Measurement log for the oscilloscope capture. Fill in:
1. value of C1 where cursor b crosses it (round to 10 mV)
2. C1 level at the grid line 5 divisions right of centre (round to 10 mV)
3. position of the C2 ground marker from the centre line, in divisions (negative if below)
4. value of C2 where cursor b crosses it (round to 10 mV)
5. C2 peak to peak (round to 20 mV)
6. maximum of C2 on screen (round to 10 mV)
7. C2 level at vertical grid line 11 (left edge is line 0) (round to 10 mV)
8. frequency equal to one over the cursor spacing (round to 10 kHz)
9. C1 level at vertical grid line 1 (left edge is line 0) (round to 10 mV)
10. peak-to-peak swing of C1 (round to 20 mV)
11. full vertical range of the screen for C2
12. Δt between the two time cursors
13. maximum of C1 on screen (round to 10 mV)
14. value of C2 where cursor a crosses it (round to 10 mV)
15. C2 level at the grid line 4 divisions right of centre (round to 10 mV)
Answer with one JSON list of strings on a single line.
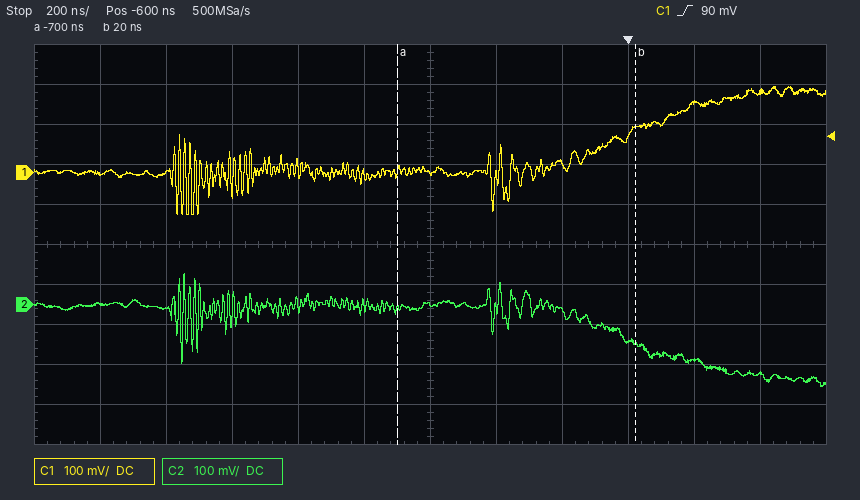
["110 mV", "200 mV", "-1.5 div", "-100 mV", "280 mV", "80 mV", "-170 mV", "1.39 MHz", "0 mV", "320 mV", "1 V", "720 ns", "220 mV", "-10 mV", "-140 mV"]
